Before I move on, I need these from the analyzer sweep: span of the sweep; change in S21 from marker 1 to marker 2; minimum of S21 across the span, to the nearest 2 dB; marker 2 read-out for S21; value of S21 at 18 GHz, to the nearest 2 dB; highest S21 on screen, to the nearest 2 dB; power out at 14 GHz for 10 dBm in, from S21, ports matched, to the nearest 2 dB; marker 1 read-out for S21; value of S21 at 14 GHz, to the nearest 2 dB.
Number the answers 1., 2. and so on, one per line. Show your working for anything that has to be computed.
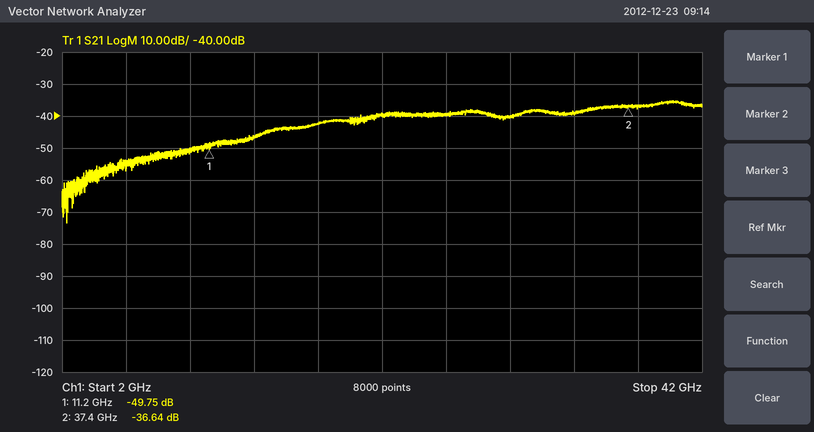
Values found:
1. 40 GHz
2. -36.64 − (-49.75) = 13.11 dB
3. -74 dB
4. -36.64 dB
5. -42 dB
6. -36 dB
7. 10 dBm + (-46 dB) = -36 dBm
8. -49.75 dB
9. -46 dB
